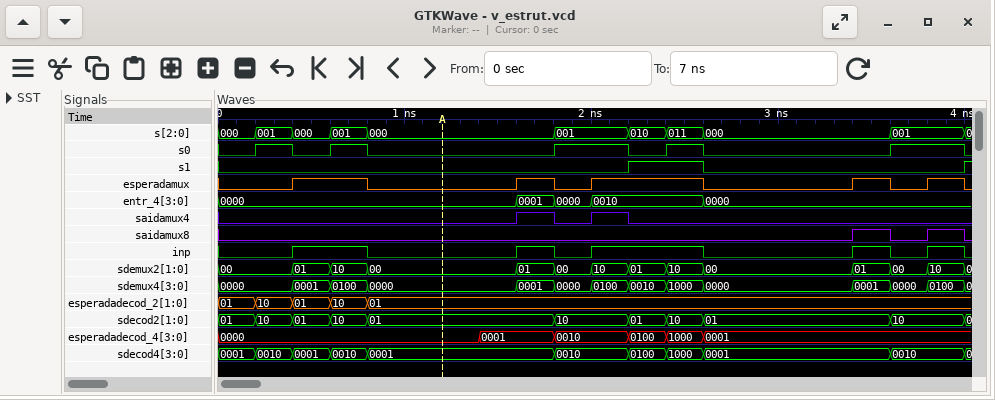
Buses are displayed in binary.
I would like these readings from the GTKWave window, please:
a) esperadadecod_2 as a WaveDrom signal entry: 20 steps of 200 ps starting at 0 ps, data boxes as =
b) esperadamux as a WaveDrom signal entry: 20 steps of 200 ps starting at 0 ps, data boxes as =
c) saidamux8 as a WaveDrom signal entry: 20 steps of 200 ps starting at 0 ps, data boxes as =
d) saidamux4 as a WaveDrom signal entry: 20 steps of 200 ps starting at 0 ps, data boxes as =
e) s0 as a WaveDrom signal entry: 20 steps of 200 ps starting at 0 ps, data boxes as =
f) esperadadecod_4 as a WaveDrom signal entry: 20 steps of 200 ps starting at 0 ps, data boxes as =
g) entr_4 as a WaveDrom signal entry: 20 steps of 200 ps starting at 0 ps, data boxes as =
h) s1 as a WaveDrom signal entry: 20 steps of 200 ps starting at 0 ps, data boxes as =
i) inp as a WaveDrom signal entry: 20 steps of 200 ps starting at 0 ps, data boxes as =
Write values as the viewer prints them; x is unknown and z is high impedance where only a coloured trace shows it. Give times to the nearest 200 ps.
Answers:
{name: 'esperadadecod_2', wave: '=====...............', data: '01 10 01 10 01'}
{name: 'esperadamux', wave: '0.1.0...101..0...101'}
{name: 'saidamux8', wave: '0................101'}
{name: 'saidamux4', wave: '0.......1010........'}
{name: 's0', wave: '01010....1.010....1.'}
{name: 'esperadadecod_4', wave: '=......=.=.===......', data: '0000 0001 0010 0100 1000 0001'}
{name: 'entr_4', wave: '=.......===..=......', data: '0000 0001 0000 0010 0000'}
{name: 's1', wave: '0..........1.0......'}
{name: 'inp', wave: '0.1.0...101..0...101'}
